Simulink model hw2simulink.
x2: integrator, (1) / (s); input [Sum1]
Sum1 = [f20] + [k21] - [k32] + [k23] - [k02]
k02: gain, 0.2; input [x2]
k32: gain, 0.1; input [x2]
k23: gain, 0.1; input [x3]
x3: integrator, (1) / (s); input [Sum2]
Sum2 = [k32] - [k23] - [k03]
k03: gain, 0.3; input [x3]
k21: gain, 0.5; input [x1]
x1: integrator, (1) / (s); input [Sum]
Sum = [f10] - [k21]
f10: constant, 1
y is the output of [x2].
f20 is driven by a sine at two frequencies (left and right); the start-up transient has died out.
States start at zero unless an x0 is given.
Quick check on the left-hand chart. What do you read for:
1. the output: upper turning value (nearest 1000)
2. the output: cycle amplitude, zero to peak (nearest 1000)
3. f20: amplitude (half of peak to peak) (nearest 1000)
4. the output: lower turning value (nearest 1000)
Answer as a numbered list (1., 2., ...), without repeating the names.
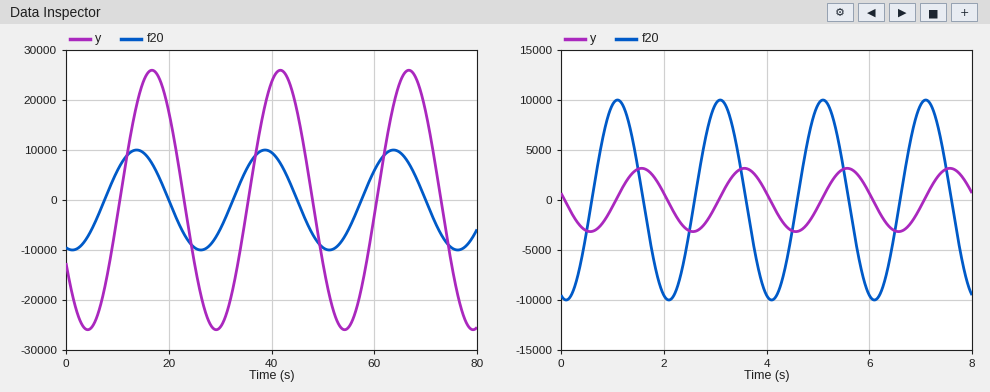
1. 26000
2. 26000
3. 10000
4. -26000
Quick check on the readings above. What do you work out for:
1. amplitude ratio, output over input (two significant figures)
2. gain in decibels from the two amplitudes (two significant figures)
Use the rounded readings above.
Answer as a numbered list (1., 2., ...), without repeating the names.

1. 2.6
2. 8.3 dB
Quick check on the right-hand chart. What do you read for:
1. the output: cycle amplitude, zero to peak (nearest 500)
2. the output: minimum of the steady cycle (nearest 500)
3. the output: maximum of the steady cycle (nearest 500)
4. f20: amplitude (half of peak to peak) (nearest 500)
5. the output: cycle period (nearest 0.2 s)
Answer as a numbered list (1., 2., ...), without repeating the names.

1. 3000
2. -3000
3. 3000
4. 10000
5. 2.0 s
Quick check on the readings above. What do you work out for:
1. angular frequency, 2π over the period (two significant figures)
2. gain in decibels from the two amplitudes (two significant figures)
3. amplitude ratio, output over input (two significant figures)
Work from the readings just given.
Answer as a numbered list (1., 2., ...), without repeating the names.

1. 3.1 rad/s
2. -10 dB
3. 0.30
